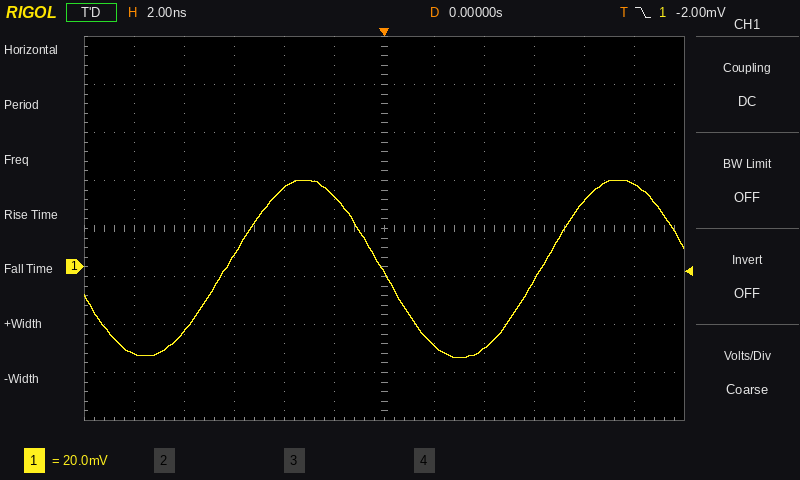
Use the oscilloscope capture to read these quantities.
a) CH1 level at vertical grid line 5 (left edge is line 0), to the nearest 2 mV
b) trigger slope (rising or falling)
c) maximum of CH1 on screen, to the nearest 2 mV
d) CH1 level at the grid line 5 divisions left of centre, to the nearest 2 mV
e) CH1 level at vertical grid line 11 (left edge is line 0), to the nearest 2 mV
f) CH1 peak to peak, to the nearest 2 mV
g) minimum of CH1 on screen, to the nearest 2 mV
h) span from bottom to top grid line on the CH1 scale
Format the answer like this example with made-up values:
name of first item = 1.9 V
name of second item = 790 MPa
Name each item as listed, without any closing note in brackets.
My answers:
CH1 level at vertical grid line 5 (left edge is line 0), to the nearest 2 mV = 30 mV
trigger slope = falling
maximum of CH1 on screen, to the nearest 2 mV = 36 mV
CH1 level at the grid line 5 divisions left of centre, to the nearest 2 mV = -36 mV
CH1 level at vertical grid line 11 (left edge is line 0), to the nearest 2 mV = 34 mV
CH1 peak to peak, to the nearest 2 mV = 74 mV
minimum of CH1 on screen, to the nearest 2 mV = -38 mV
span from bottom to top grid line on the CH1 scale = 160 mV
